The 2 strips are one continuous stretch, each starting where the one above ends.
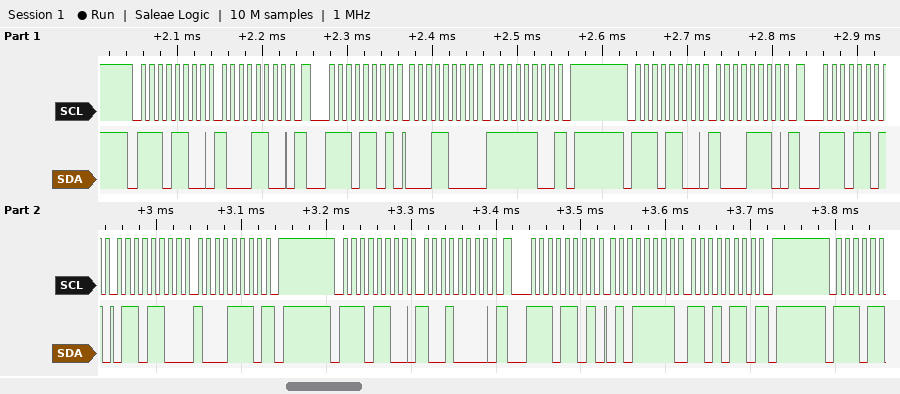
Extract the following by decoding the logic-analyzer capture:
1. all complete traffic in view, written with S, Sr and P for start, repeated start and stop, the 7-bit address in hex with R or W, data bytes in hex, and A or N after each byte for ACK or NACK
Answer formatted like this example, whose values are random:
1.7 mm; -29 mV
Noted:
S 76W A 8C A Sr 76R A 18 A FC N P S 76W A 8E A Sr 76R A 6C A 8E N P S 76W A 90 A Sr 76R A 5F A D6 N P
